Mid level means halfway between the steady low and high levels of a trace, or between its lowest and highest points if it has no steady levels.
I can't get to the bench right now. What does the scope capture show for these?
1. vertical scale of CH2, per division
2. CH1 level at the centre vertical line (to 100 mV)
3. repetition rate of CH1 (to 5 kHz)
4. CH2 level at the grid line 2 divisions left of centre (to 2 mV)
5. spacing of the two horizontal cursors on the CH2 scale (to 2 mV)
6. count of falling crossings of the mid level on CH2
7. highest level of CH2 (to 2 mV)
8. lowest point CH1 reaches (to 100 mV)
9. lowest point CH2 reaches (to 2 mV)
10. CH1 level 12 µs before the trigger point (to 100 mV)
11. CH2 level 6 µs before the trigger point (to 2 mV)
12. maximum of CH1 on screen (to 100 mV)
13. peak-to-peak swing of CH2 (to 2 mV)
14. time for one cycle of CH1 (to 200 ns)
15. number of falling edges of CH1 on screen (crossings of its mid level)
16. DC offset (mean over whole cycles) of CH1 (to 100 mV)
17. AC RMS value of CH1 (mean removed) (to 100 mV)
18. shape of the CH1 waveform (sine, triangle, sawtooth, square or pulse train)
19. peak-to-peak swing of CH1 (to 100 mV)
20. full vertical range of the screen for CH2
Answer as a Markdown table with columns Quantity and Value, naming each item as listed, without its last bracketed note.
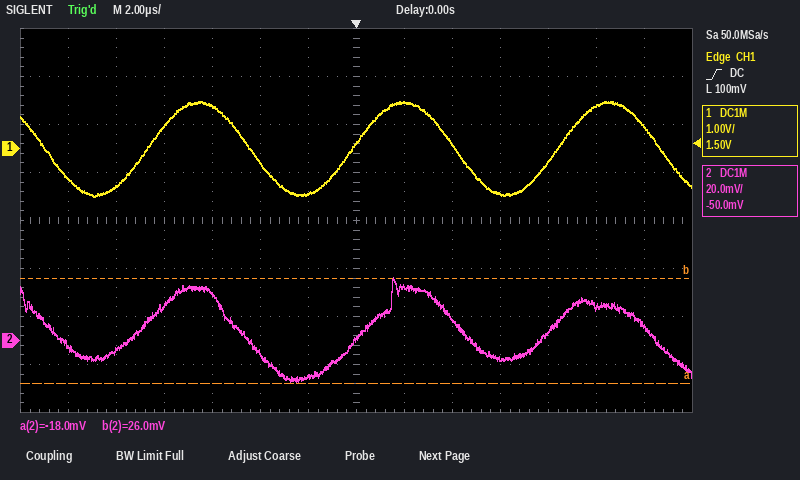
| Quantity | Value |
|---|---|
| vertical scale of CH2, per division | 20 mV |
| CH1 level at the centre vertical line | 100 mV |
| repetition rate of CH1 | 115 kHz |
| CH2 level at the grid line 2 divisions left of centre | -6 mV |
| spacing of the two horizontal cursors on the CH2 scale | 44 mV |
| count of falling crossings of the mid level on CH2 | 4 |
| highest level of CH2 | 26 mV |
| lowest point CH1 reaches | -1.0 V |
| lowest point CH2 reaches | -18 mV |
| CH1 level 12 µs before the trigger point | -600 mV |
| CH2 level 6 µs before the trigger point | 20 mV |
| maximum of CH1 on screen | 1.0 V |
| peak-to-peak swing of CH2 | 44 mV |
| time for one cycle of CH1 | 8.6 µs |
| number of falling edges of CH1 on screen | 4 |
| DC offset (mean over whole cycles) of CH1 | 0.0 V |
| AC RMS value of CH1 (mean removed) | 700 mV |
| shape of the CH1 waveform | sine |
| peak-to-peak swing of CH1 | 2.0 V |
| full vertical range of the screen for CH2 | 160 mV |
